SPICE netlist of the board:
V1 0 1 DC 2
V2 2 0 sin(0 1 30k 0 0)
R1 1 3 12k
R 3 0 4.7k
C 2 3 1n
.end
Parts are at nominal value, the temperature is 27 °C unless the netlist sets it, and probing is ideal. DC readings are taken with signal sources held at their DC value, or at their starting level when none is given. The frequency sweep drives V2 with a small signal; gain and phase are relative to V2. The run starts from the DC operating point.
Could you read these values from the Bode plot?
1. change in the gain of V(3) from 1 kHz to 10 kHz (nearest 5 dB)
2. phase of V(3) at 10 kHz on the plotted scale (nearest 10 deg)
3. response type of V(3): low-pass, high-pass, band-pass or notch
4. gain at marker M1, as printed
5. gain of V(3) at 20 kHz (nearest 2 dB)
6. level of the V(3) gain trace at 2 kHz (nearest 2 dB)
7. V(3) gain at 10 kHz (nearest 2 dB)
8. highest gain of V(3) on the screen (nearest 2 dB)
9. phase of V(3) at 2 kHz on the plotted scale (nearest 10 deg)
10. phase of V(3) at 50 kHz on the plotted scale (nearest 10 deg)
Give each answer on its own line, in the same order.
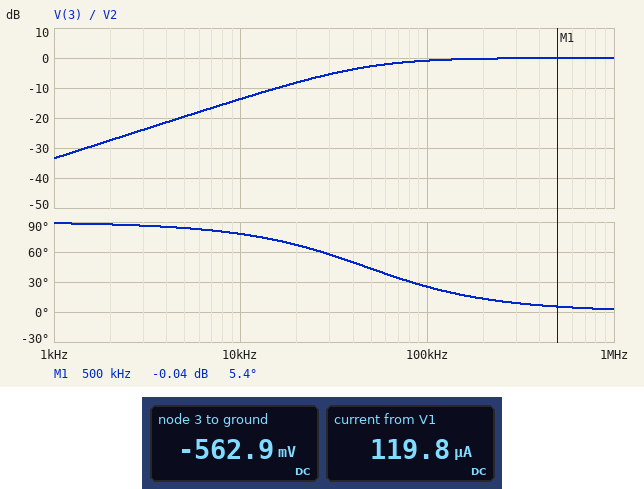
20 dB
80 deg
high-pass
-0.04 dB
-8 dB
-28 dB
-14 dB
0 dB
90 deg
40 deg
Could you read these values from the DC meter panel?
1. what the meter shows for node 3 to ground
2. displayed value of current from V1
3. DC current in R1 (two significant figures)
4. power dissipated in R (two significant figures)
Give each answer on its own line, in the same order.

-562.9 mV
119.8 µA
120 µA
67 µW
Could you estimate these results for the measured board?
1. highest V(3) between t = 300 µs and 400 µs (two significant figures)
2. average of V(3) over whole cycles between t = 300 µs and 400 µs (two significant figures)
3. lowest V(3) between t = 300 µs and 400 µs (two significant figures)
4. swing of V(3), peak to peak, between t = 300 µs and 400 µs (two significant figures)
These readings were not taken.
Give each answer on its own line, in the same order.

-26 mV
-560 mV
-1.1 V
1.1 V
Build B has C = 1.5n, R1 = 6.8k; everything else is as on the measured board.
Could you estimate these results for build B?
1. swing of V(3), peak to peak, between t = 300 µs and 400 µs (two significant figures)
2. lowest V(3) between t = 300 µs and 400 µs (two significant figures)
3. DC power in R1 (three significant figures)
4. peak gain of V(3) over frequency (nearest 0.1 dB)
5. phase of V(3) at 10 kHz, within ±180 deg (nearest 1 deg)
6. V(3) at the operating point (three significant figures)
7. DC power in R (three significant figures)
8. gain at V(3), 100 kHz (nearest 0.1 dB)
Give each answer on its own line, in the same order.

1.2 V
-1.4 V
206 µW
0 dB
75 deg
-817 mV
142 µW
-0.6 dB
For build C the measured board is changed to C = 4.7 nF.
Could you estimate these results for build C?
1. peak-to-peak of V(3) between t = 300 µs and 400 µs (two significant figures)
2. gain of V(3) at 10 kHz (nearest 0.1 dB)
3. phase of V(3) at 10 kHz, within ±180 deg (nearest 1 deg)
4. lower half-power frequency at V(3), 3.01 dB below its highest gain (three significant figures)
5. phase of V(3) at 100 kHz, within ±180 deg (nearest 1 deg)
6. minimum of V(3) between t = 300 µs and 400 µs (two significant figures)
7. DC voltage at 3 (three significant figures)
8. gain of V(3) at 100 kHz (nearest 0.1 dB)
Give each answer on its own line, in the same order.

1.9 V
-3.0 dB
45 deg
10.0 kHz
6 deg
-1.5 V
-563 mV
0 dB
